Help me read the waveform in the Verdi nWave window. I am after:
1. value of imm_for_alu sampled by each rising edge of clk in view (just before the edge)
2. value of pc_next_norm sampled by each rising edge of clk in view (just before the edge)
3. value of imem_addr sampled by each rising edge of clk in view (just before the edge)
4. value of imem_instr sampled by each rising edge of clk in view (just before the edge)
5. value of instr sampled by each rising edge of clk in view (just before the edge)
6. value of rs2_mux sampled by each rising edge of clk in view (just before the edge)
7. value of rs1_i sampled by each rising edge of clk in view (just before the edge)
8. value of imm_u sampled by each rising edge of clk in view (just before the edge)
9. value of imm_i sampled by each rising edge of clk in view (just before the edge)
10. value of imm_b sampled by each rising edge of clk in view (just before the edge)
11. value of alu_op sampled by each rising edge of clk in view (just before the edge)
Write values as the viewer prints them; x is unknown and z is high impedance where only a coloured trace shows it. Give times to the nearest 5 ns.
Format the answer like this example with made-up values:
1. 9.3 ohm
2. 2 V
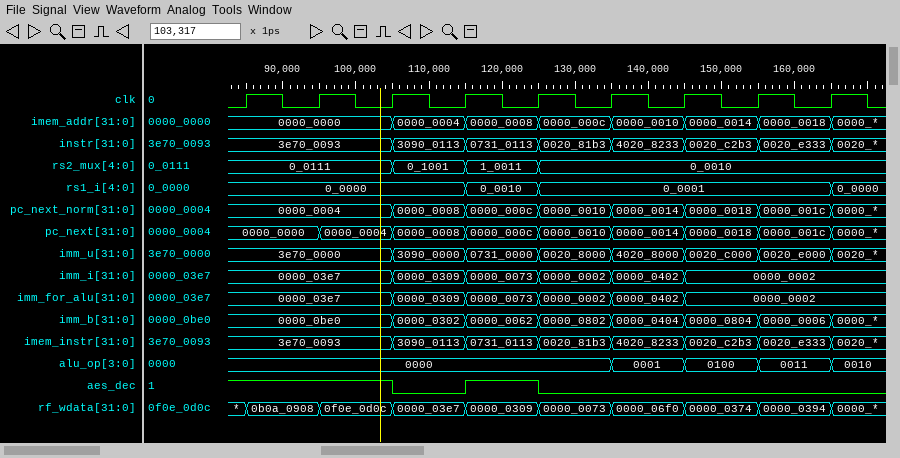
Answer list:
1. 0000_03e7, 0000_03e7, 0000_03e7, 0000_0309, 0000_0073, 0000_0002, 0000_0402, 0000_0002, 0000_0002
2. 0000_0004, 0000_0004, 0000_0004, 0000_0008, 0000_000c, 0000_0010, 0000_0014, 0000_0018, 0000_001c
3. 0000_0000, 0000_0000, 0000_0000, 0000_0004, 0000_0008, 0000_000c, 0000_0010, 0000_0014, 0000_0018
4. 3e70_0093, 3e70_0093, 3e70_0093, 3090_0113, 0731_0113, 0020_81b3, 4020_8233, 0020_c2b3, 0020_e333
5. 3e70_0093, 3e70_0093, 3e70_0093, 3090_0113, 0731_0113, 0020_81b3, 4020_8233, 0020_c2b3, 0020_e333
6. 0_0111, 0_0111, 0_0111, 0_1001, 1_0011, 0_0010, 0_0010, 0_0010, 0_0010
7. 0_0000, 0_0000, 0_0000, 0_0000, 0_0010, 0_0001, 0_0001, 0_0001, 0_0001
8. 3e70_0000, 3e70_0000, 3e70_0000, 3090_0000, 0731_0000, 0020_8000, 4020_8000, 0020_c000, 0020_e000
9. 0000_03e7, 0000_03e7, 0000_03e7, 0000_0309, 0000_0073, 0000_0002, 0000_0402, 0000_0002, 0000_0002
10. 0000_0be0, 0000_0be0, 0000_0be0, 0000_0302, 0000_0062, 0000_0802, 0000_0404, 0000_0804, 0000_0006
11. 0000, 0000, 0000, 0000, 0000, 0000, 0001, 0100, 0011
